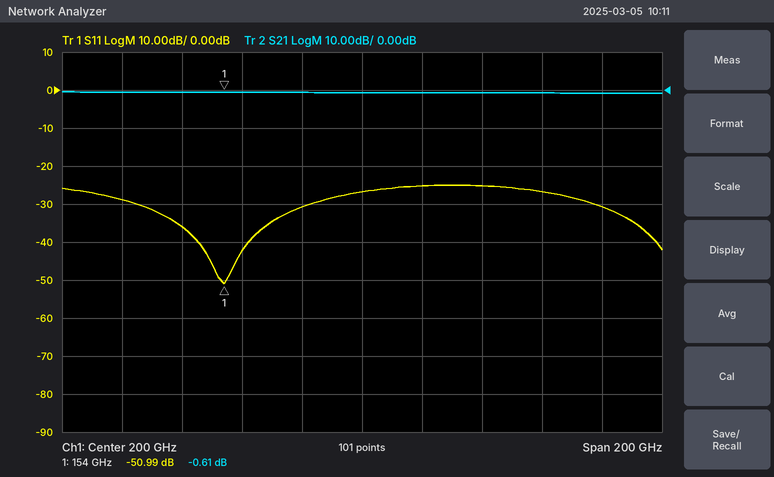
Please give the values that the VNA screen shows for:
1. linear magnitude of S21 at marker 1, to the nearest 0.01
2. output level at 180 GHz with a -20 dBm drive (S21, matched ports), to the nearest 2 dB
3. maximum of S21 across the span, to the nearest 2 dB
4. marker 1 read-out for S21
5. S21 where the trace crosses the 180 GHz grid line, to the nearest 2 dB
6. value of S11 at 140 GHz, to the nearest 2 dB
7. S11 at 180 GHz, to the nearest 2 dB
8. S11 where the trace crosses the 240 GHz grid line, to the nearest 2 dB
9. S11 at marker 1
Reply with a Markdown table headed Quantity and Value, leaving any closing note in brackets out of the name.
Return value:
| Quantity | Value |
|---|---|
| linear magnitude of S21 at marker 1, to the nearest 0.01 | 0.93 |
| output level at 180 GHz with a -20 dBm drive (S21, matched ports), to the nearest 2 dB | -20 dBm |
| maximum of S21 across the span, to the nearest 2 dB | 0 dB |
| marker 1 read-out for S21 | -0.61 dB |
| S21 where the trace crosses the 180 GHz grid line, to the nearest 2 dB | 0 dB |
| value of S11 at 140 GHz, to the nearest 2 dB | -36 dB |
| S11 at 180 GHz, to the nearest 2 dB | -30 dB |
| S11 where the trace crosses the 240 GHz grid line, to the nearest 2 dB | -26 dB |
| S11 at marker 1 | -50.99 dB |
